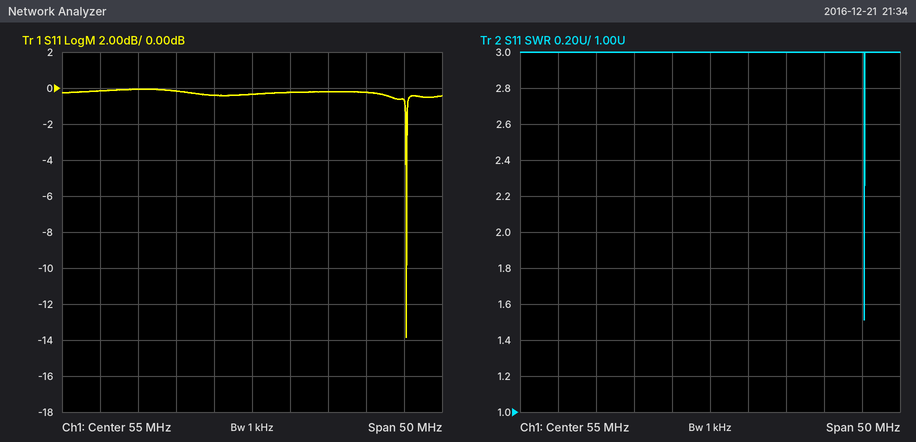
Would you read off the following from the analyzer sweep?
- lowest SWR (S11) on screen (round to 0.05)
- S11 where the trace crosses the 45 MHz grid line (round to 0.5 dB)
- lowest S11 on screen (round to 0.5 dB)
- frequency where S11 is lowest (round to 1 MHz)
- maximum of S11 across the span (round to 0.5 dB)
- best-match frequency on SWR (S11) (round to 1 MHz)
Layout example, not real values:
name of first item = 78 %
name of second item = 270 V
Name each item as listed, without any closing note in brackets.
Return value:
lowest SWR (S11) on screen = 1.50
S11 where the trace crosses the 45 MHz grid line = 0.0 dB
lowest S11 on screen = -14.0 dB
frequency where S11 is lowest = 75 MHz
maximum of S11 across the span = 0.0 dB
best-match frequency on SWR (S11) = 75 MHz
